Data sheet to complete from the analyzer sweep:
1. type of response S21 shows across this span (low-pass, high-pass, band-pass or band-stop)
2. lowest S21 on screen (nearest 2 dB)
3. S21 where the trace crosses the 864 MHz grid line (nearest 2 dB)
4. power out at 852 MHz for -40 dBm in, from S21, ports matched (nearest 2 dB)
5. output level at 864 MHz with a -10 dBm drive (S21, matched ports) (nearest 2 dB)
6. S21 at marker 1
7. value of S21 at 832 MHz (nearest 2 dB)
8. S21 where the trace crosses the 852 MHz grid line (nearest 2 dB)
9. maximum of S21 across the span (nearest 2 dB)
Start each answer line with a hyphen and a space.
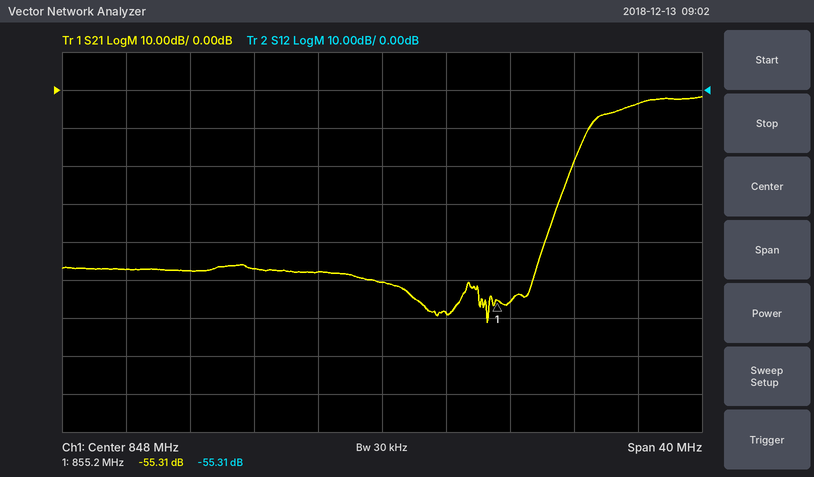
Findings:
- high-pass
- -62 dB
- -4 dB
- -98 dBm
- -14 dBm
- -55.31 dB
- -48 dB
- -58 dB
- -2 dB
